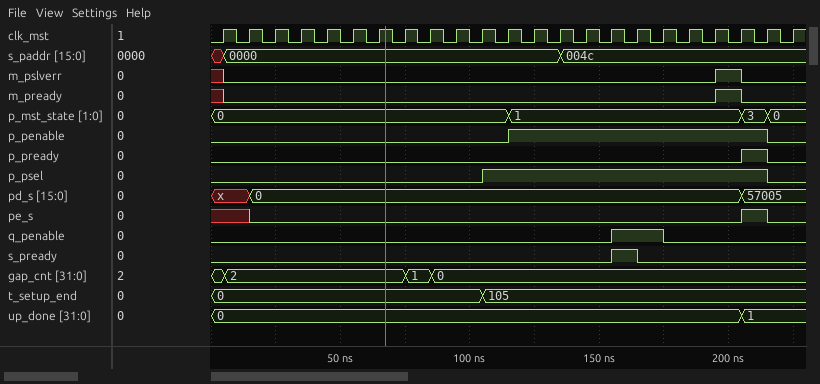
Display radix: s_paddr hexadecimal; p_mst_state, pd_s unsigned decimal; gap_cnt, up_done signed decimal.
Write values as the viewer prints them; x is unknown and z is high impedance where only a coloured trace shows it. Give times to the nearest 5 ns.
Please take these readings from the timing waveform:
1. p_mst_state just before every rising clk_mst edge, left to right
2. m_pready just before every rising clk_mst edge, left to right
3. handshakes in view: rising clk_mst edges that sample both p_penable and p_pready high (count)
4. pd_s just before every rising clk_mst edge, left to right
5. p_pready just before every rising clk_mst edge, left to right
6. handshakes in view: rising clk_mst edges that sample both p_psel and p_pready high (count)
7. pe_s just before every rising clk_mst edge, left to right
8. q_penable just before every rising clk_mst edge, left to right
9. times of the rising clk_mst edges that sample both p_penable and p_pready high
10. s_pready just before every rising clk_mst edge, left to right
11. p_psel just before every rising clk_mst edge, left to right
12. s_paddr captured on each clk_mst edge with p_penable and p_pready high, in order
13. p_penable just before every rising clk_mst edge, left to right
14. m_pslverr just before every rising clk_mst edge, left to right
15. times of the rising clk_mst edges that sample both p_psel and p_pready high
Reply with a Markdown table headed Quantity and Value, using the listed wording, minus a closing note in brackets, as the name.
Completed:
| Quantity | Value |
|---|---|
| p_mst_state just before every rising clk_mst edge, left to right | 0, 0, 0, 0, 0, 0, 0, 0, 0, 0, 0, 0, 1, 1, 1, 1, 1, 1, 1, 1, 1, 3, 0 |
| m_pready just before every rising clk_mst edge, left to right | x 0 0 0 0 0 0 0 0 0 0 0 0 0 0 0 0 0 0 0 1 0 0 |
| handshakes in view: rising clk_mst edges that sample both p_penable and p_pready high | 1 |
| pd_s just before every rising clk_mst edge, left to right | x, x, 0, 0, 0, 0, 0, 0, 0, 0, 0, 0, 0, 0, 0, 0, 0, 0, 0, 0, 0, 57005, 57005 |
| p_pready just before every rising clk_mst edge, left to right | 0 0 0 0 0 0 0 0 0 0 0 0 0 0 0 0 0 0 0 0 0 1 0 |
| handshakes in view: rising clk_mst edges that sample both p_psel and p_pready high | 1 |
| pe_s just before every rising clk_mst edge, left to right | x x 0 0 0 0 0 0 0 0 0 0 0 0 0 0 0 0 0 0 0 1 0 |
| q_penable just before every rising clk_mst edge, left to right | 0 0 0 0 0 0 0 0 0 0 0 0 0 0 0 0 1 1 0 0 0 0 0 |
| times of the rising clk_mst edges that sample both p_penable and p_pready high | 215 ns |
| s_pready just before every rising clk_mst edge, left to right | 0 0 0 0 0 0 0 0 0 0 0 0 0 0 0 0 1 0 0 0 0 0 0 |
| p_psel just before every rising clk_mst edge, left to right | 0 0 0 0 0 0 0 0 0 0 0 1 1 1 1 1 1 1 1 1 1 1 0 |
| s_paddr captured on each clk_mst edge with p_penable and p_pready high, in order | 004c |
| p_penable just before every rising clk_mst edge, left to right | 0 0 0 0 0 0 0 0 0 0 0 0 1 1 1 1 1 1 1 1 1 1 0 |
| m_pslverr just before every rising clk_mst edge, left to right | x 0 0 0 0 0 0 0 0 0 0 0 0 0 0 0 0 0 0 0 1 0 0 |
| times of the rising clk_mst edges that sample both p_psel and p_pready high | 215 ns |
